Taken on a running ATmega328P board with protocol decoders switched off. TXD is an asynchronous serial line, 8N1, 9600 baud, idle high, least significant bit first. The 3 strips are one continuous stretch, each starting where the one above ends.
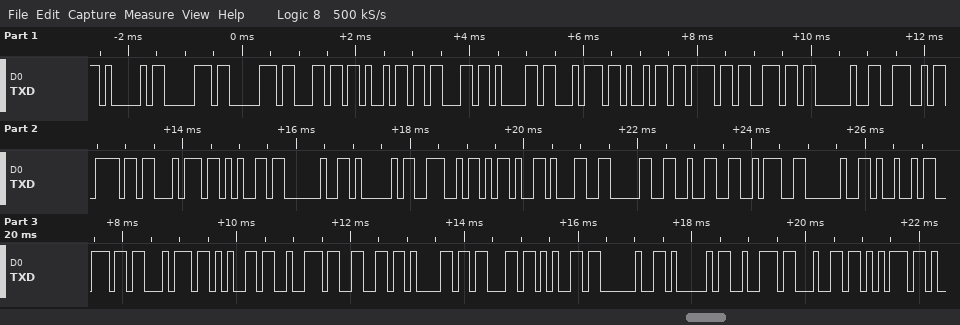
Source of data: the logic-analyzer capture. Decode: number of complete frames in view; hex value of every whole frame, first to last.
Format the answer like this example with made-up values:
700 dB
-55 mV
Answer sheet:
39
41 70 70 6C 69 63 61 74 69 6F 6E 20 4E 6F 74 65 20 41 4E 2D 31 30 32 3A 20 49 6E 74 65 72 66 61 63 65 20 41 72 64 75
